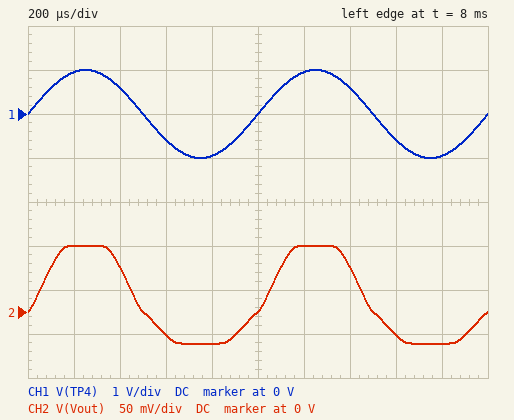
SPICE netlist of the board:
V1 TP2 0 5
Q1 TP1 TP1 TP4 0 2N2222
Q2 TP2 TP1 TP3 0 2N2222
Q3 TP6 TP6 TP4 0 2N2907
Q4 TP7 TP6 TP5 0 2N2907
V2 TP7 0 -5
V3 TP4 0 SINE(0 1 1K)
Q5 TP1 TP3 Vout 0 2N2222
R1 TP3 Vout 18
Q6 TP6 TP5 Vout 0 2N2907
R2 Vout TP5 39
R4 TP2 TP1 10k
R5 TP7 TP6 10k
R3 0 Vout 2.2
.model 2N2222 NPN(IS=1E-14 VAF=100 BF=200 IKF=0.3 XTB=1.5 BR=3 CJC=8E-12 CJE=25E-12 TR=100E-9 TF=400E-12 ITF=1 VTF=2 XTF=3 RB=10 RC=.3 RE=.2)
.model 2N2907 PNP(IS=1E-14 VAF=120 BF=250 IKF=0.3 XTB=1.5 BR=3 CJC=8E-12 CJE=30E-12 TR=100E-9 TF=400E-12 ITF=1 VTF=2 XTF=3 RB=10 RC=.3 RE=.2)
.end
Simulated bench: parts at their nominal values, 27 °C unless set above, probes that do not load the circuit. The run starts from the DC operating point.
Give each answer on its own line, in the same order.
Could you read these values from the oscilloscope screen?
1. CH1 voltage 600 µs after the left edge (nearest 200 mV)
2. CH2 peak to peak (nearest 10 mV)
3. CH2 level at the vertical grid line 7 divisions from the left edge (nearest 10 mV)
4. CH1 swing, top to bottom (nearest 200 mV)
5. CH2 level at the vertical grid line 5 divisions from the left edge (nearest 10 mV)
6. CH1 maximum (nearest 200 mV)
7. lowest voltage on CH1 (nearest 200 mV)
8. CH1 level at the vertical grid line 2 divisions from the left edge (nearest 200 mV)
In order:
-600 mV
110 mV
50 mV
2.0 V
0 V
1.0 V
-1.0 V
600 mV
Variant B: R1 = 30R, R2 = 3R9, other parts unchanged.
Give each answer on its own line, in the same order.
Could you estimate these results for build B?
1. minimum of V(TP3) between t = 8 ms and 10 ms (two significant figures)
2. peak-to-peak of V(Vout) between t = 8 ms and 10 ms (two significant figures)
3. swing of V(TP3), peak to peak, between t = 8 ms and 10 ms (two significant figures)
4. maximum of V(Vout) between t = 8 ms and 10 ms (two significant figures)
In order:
-170 mV
220 mV
840 mV
46 mV
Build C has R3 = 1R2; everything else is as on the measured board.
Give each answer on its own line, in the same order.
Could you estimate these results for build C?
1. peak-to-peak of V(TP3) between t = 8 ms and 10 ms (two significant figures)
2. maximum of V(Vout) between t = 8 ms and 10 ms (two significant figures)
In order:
670 mV
41 mV
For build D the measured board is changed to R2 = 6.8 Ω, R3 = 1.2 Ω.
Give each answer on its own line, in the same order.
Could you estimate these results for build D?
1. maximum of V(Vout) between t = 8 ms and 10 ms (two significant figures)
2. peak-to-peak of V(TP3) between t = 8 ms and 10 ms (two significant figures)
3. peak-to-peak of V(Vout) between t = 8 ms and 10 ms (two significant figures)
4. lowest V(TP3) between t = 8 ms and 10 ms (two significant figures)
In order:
41 mV
740 mV
130 mV
-90 mV
